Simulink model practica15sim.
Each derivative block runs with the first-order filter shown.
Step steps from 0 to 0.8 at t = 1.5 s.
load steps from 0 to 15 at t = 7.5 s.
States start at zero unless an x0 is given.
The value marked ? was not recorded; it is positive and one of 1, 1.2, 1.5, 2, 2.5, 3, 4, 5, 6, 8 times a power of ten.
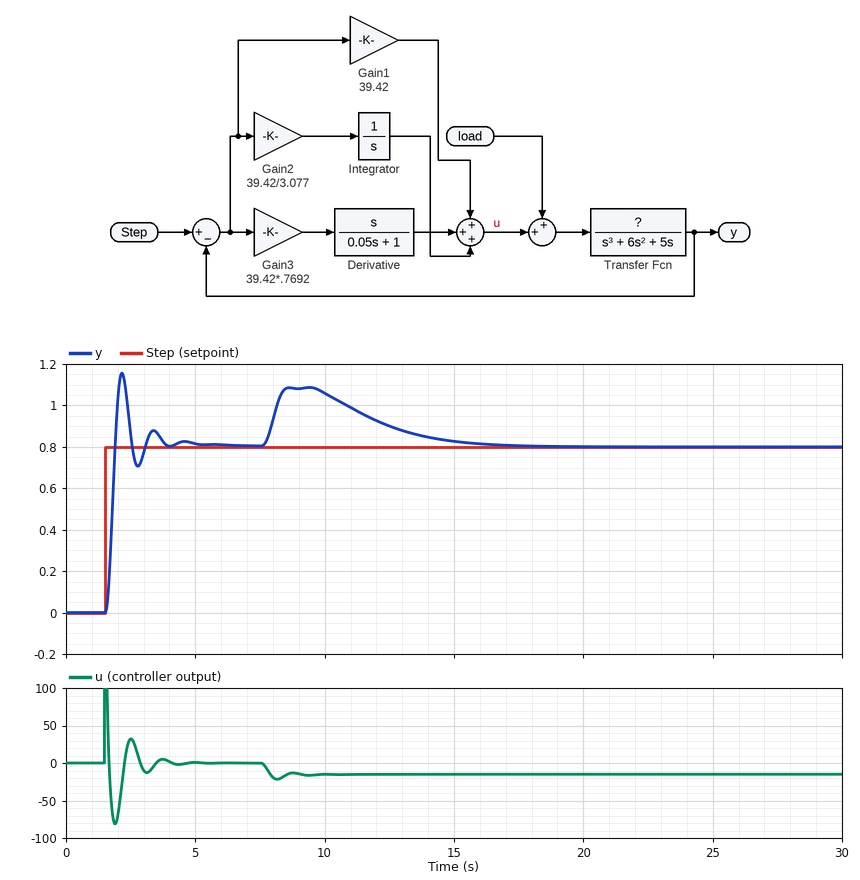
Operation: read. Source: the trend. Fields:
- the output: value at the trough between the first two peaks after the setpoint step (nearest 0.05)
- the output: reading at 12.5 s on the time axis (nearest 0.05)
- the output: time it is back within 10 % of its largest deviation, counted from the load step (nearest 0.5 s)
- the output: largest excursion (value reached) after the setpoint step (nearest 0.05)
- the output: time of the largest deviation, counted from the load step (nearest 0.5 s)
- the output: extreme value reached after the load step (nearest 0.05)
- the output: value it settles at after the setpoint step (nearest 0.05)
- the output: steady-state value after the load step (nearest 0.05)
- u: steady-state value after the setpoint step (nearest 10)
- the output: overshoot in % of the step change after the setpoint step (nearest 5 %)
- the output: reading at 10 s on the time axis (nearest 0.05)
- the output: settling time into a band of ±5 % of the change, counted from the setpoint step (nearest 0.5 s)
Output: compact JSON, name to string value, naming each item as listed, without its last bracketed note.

{"the output: value at the trough between the first two peaks after the setpoint step": "0.70", "the output: reading at 12.5 s on the time axis": "0.90", "the output: time it is back within 10 % of its largest deviation, counted from the load step": "7.5 s", "the output: largest excursion (value reached) after the setpoint step": "1.15", "the output: time of the largest deviation, counted from the load step": "2.0 s", "the output: extreme value reached after the load step": "1.10", "the output: value it settles at after the setpoint step": "0.80", "the output: steady-state value after the load step": "0.80", "u: steady-state value after the setpoint step": "0", "the output: overshoot in % of the step change after the setpoint step": "45 %", "the output: reading at 10 s on the time axis": "1.05", "the output: settling time into a band of ±5 % of the change, counted from the setpoint step": "2.0 s"}
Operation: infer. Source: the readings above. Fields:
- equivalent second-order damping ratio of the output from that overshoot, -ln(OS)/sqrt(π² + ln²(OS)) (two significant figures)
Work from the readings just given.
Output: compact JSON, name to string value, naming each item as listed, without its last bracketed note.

{"equivalent second-order damping ratio of the output from that overshoot, -ln(OS)/sqrt(π² + ln²(OS))": "0.25"}
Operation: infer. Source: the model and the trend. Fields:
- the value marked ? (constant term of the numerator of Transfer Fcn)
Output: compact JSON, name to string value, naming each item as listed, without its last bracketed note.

{"the value marked ?": "1"}
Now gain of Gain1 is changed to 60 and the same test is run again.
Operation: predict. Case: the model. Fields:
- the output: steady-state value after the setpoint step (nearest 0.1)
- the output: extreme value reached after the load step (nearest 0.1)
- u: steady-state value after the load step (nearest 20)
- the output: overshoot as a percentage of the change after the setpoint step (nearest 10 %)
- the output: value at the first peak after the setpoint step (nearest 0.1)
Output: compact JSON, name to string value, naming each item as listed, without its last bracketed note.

{"the output: steady-state value after the setpoint step": "0.8", "the output: extreme value reached after the load step": "1.0", "u: steady-state value after the load step": "-20", "the output: overshoot as a percentage of the change after the setpoint step": "60 %", "the output: value at the first peak after the setpoint step": "1.3"}
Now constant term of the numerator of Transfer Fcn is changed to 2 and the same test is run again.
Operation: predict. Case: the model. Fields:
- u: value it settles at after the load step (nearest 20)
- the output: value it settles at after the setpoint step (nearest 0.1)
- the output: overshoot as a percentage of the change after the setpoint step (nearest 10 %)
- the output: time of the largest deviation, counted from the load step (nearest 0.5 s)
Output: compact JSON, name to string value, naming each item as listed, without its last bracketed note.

{"u: value it settles at after the load step": "-20", "the output: value it settles at after the setpoint step": "0.8", "the output: overshoot as a percentage of the change after the setpoint step": "70 %", "the output: time of the largest deviation, counted from the load step": "1.5 s"}
